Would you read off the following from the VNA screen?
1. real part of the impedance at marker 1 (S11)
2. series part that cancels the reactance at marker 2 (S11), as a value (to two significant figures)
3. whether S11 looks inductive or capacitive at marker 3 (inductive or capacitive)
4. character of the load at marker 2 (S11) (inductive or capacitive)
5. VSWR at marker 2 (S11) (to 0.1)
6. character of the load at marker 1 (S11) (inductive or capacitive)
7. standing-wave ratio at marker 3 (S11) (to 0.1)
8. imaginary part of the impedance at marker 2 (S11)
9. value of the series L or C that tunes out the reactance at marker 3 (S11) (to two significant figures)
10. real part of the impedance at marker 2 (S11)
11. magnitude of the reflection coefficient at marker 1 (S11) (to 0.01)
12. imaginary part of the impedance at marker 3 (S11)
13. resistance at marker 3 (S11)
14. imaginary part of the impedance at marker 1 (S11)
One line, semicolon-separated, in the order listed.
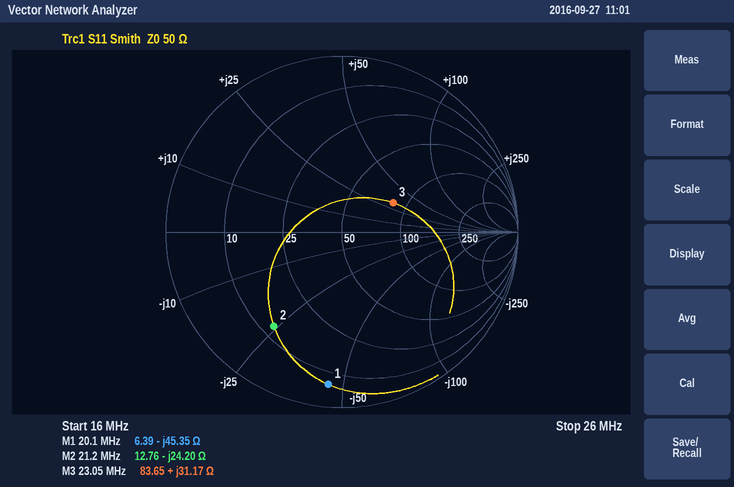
6.39 Ω; 180 nH; inductive; capacitive; 4.9; capacitive; 2.0; -24.20 Ω; 220 pF; 12.76 Ω; 0.87; +31.17 Ω; 83.65 Ω; -45.35 Ω
